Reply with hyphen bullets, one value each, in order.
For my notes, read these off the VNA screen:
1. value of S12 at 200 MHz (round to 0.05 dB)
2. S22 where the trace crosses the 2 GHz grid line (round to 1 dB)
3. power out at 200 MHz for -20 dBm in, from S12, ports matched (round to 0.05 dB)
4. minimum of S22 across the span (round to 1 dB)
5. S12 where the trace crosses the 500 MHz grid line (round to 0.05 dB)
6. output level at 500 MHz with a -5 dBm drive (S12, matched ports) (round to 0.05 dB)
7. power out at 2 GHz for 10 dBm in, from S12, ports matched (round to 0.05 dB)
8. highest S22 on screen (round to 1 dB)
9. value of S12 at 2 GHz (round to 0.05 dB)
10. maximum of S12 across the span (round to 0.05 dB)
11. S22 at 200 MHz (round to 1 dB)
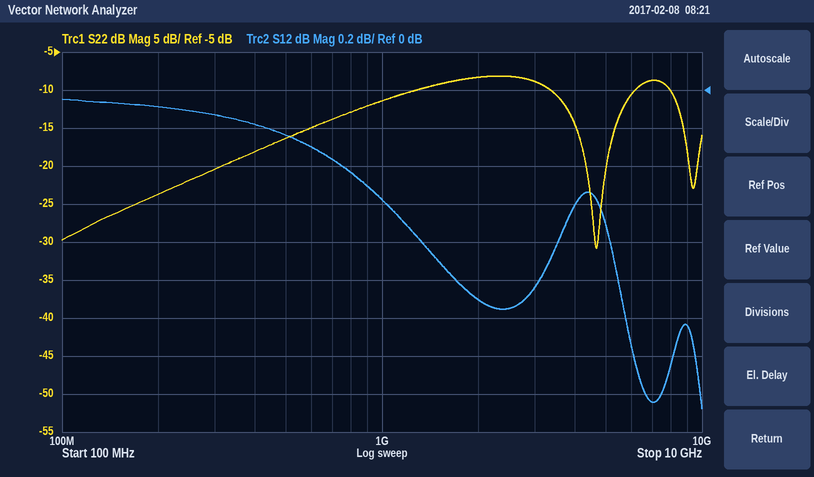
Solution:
- -0.10 dB
- -8 dB
- -20.10 dBm
- -31 dB
- -0.25 dB
- -5.25 dBm
- 8.90 dBm
- -8 dB
- -1.10 dB
- -0.05 dB
- -24 dB
